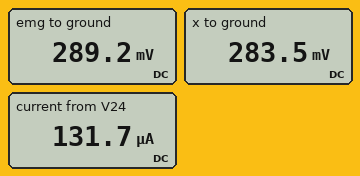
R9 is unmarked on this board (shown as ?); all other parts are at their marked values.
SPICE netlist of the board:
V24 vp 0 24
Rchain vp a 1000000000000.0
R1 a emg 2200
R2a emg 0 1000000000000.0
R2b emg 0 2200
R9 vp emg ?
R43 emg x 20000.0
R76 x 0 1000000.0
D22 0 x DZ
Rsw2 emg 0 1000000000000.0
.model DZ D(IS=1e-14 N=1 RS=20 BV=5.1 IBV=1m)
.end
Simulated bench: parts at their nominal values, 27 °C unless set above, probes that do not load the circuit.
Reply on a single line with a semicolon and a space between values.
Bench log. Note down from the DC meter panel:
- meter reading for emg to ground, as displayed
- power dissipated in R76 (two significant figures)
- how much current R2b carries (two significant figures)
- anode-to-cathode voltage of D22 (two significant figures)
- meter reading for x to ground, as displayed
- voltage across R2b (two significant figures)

289.2 mV; 80 nW; 130 µA; -280 mV; 283.5 mV; 290 mV
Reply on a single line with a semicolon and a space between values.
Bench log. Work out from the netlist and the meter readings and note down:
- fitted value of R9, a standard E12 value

180 kΩ
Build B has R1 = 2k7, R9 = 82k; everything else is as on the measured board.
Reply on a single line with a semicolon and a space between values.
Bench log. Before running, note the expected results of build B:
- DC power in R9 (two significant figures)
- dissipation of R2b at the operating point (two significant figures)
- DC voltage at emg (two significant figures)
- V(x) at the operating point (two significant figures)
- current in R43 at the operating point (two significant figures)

6.7 mW; 180 µW; 630 mV; 610 mV; 610 nA
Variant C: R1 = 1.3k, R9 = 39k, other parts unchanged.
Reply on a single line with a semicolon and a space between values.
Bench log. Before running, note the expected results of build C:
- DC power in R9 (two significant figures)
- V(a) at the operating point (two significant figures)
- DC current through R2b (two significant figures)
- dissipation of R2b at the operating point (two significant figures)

13 mW; 1.3 V; 580 µA; 740 µW
